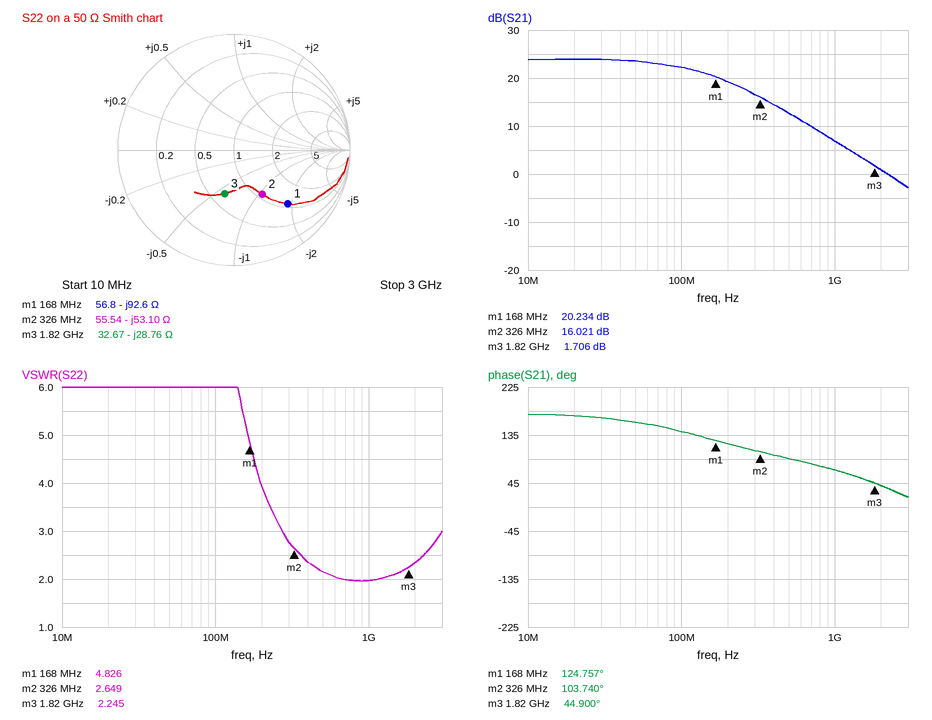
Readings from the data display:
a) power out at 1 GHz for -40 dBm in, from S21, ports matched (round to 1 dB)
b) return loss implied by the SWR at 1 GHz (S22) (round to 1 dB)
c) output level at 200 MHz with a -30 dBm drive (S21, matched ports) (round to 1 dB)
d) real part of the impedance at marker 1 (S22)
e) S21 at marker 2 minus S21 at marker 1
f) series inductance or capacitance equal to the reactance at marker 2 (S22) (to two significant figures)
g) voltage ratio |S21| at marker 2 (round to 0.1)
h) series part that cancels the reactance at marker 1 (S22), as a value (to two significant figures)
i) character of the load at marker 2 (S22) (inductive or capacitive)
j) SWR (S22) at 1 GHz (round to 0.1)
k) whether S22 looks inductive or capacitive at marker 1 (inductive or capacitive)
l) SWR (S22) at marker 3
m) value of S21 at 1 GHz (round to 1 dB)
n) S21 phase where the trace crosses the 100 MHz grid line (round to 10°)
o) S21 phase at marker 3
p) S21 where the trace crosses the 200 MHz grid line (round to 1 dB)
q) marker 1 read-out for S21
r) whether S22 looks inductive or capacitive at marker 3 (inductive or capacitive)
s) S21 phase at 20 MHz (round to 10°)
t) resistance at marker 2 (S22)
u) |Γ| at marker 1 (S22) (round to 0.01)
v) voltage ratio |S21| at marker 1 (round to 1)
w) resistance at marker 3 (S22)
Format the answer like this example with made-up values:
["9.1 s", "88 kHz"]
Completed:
["-33 dBm", "10 dB", "-11 dBm", "56.8 Ω", "-4.213 dB", "9.2 pF", "6.3", "88 nH", "capacitive", "2.0", "capacitive", "2.245", "7 dB", "140°", "44.900°", "19 dB", "20.234 dB", "capacitive", "170°", "55.54 Ω", "0.66", "10", "32.67 Ω"]
